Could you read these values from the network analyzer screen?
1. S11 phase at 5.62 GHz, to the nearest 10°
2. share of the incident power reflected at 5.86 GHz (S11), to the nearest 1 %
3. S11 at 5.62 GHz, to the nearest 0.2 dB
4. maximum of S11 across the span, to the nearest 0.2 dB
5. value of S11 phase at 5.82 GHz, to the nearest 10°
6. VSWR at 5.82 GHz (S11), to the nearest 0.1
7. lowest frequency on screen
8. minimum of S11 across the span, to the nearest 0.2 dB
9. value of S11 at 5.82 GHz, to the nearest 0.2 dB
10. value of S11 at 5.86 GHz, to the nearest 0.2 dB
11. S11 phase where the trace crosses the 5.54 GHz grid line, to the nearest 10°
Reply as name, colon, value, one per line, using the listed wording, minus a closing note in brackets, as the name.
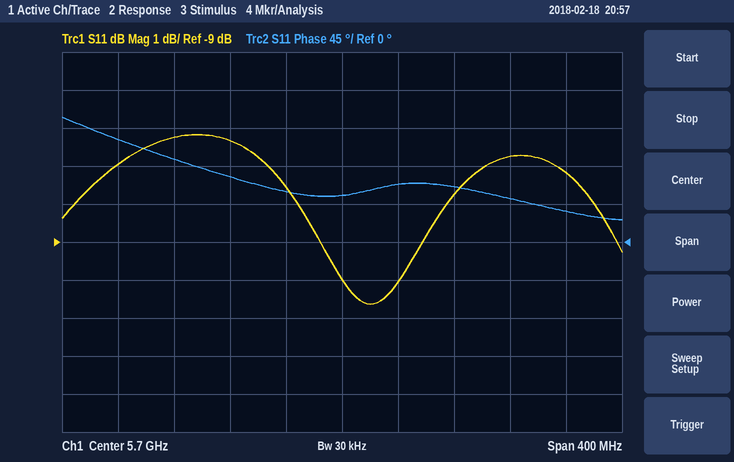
S11 phase at 5.62 GHz, to the nearest 10°: 80°
share of the incident power reflected at 5.86 GHz (S11), to the nearest 1 %: 19 %
S11 at 5.62 GHz, to the nearest 0.2 dB: -6.4 dB
maximum of S11 across the span, to the nearest 0.2 dB: -6.2 dB
value of S11 phase at 5.82 GHz, to the nearest 10°: 50°
VSWR at 5.82 GHz (S11), to the nearest 0.1: 2.7
lowest frequency on screen: 5.5 GHz
minimum of S11 across the span, to the nearest 0.2 dB: -10.6 dB
value of S11 at 5.82 GHz, to the nearest 0.2 dB: -6.8 dB
value of S11 at 5.86 GHz, to the nearest 0.2 dB: -7.2 dB
S11 phase where the trace crosses the 5.54 GHz grid line, to the nearest 10°: 120°
